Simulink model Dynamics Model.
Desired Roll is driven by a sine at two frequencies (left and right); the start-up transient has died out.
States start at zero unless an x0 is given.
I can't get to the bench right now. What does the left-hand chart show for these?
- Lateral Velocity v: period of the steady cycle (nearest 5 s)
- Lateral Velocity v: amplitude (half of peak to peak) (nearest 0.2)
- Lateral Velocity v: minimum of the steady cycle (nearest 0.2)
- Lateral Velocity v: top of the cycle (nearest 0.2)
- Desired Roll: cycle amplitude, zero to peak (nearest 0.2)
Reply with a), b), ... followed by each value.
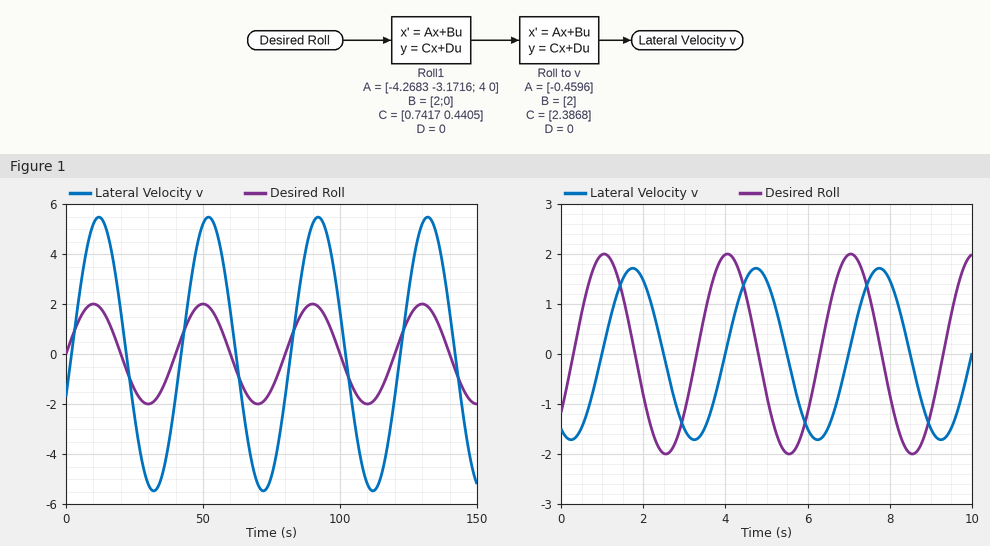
a) 40 s
b) 5.4
c) -5.4
d) 5.4
e) 2.0
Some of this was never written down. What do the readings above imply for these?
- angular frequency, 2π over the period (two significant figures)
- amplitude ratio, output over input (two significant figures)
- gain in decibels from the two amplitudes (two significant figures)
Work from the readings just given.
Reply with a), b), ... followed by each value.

a) 0.16 rad/s
b) 2.7
c) 8.6 dB
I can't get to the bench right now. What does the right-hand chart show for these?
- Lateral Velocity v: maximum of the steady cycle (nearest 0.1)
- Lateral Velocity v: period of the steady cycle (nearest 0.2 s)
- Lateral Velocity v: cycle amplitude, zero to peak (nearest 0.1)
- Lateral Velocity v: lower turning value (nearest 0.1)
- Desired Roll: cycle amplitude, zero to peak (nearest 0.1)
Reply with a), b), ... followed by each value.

a) 1.7
b) 3.0 s
c) 1.7
d) -1.7
e) 2.0
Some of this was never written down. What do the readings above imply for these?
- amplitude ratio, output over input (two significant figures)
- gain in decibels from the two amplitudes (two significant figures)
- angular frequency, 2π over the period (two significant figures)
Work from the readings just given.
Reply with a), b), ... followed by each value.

a) 0.85
b) -1.4 dB
c) 2.1 rad/s
